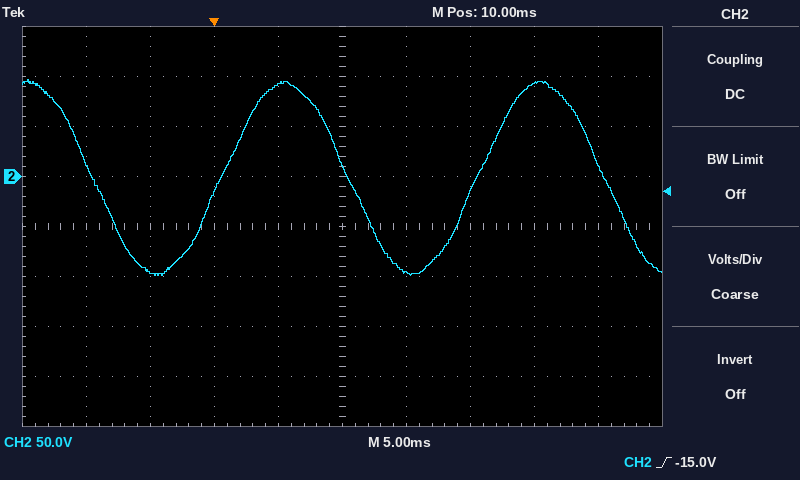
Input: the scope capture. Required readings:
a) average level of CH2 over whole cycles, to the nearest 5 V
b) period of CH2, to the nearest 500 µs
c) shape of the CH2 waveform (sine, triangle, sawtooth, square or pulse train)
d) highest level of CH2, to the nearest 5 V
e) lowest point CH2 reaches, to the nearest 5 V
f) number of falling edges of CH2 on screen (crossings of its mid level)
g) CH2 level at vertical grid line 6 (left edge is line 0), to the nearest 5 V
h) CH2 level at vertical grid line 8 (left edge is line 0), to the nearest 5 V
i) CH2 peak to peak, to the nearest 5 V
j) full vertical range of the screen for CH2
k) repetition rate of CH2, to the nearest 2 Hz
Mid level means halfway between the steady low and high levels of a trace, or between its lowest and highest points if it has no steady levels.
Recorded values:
0 V
20.0 ms
sine
95 V
-100 V
3
-95 V
95 V
195 V
400 V
50 Hz
